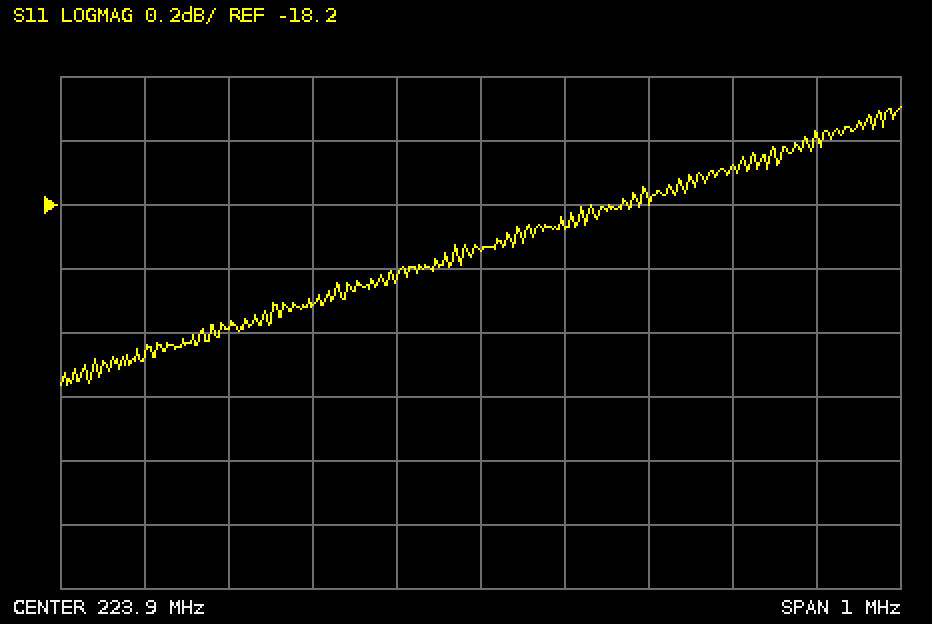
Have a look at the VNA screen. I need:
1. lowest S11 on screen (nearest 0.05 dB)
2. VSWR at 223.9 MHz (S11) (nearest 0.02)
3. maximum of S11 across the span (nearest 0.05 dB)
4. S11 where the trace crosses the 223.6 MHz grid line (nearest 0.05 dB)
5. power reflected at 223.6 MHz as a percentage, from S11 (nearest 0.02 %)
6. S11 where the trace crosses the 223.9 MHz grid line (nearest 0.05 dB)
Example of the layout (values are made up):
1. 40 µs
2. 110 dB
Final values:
1. -18.75 dB
2. 1.28
3. -17.90 dB
4. -18.60 dB
5. 1.38 %
6. -18.35 dB
